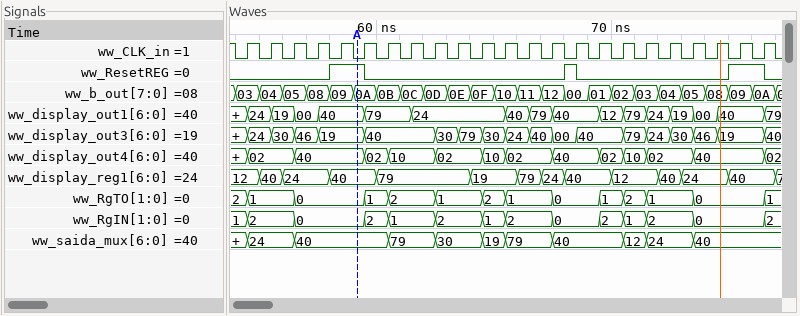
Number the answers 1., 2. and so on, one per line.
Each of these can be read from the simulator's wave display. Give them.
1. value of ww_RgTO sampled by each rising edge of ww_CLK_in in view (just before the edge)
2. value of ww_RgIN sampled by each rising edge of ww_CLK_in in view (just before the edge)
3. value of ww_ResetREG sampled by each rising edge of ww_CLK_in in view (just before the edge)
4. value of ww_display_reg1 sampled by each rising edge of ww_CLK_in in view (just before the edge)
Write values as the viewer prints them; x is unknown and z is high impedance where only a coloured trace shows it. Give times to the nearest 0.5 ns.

1. 2, 1, 1, 0, 0, 0, 1, 2, 2, 1, 1, 2, 1, 1, 0, 0, 1, 2, 1, 1, 0, 0, 0
2. 1, 2, 2, 0, 0, 0, 2, 1, 1, 2, 2, 1, 2, 2, 0, 0, 2, 1, 2, 2, 0, 0, 0
3. 0 0 0 0 1 1 0 0 0 0 0 0 0 0 1 0 0 0 0 0 0 1 1
4. 12, 40, 24, 24, 40, 40, 79, 79, 79, 79, 19, 19, 79, 24, 40, 40, 12, 12, 40, 24, 24, 40, 40
